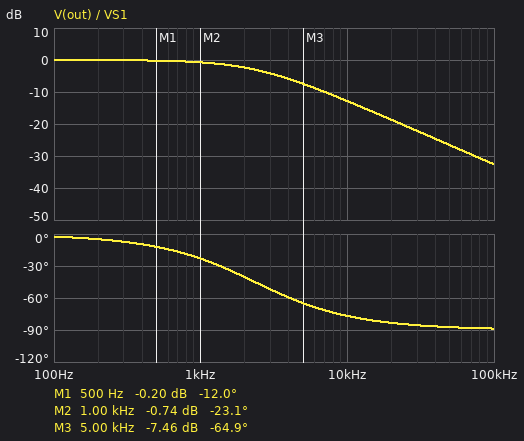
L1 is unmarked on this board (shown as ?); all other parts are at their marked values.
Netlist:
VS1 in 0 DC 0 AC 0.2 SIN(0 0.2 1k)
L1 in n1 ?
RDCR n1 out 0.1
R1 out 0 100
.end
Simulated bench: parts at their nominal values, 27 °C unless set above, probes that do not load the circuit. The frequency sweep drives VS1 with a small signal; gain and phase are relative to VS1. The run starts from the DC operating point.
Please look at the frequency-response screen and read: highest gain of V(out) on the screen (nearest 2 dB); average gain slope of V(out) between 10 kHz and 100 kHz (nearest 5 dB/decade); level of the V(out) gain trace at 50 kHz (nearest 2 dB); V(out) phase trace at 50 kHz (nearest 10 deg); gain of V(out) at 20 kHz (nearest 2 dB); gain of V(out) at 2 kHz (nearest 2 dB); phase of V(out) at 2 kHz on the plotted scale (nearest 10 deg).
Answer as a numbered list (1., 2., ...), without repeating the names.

1. 0 dB
2. -20 dB/decade
3. -26 dB
4. -90 deg
5. -18 dB
6. -2 dB
7. -40 deg
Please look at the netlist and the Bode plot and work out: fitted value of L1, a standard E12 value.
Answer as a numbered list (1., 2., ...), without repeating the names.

1. 6.8 mH
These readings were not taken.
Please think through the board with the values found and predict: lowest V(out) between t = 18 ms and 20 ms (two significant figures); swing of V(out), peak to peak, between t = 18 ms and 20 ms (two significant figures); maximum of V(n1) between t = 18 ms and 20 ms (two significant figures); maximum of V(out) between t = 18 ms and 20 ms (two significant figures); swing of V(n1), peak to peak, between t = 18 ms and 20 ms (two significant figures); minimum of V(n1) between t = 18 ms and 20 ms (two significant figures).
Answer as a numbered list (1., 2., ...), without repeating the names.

1. -180 mV
2. 370 mV
3. 180 mV
4. 180 mV
5. 370 mV
6. -180 mV
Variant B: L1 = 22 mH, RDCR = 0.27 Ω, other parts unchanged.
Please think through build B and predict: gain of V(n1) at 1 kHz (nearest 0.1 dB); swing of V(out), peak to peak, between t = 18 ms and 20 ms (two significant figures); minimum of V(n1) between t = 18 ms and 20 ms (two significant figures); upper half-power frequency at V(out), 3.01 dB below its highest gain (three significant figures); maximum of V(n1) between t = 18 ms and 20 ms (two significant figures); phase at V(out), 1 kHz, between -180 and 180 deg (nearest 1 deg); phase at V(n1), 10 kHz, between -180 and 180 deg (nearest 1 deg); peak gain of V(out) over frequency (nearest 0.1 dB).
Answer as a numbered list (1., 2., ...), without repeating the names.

1. -4.6 dB
2. 230 mV
3. -120 mV
4. 725 Hz
5. 120 mV
6. -54 deg
7. -86 deg
8. 0 dB
